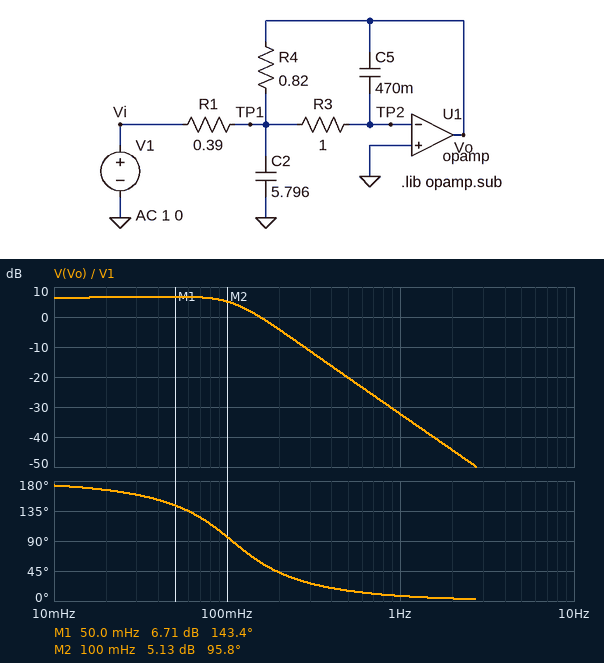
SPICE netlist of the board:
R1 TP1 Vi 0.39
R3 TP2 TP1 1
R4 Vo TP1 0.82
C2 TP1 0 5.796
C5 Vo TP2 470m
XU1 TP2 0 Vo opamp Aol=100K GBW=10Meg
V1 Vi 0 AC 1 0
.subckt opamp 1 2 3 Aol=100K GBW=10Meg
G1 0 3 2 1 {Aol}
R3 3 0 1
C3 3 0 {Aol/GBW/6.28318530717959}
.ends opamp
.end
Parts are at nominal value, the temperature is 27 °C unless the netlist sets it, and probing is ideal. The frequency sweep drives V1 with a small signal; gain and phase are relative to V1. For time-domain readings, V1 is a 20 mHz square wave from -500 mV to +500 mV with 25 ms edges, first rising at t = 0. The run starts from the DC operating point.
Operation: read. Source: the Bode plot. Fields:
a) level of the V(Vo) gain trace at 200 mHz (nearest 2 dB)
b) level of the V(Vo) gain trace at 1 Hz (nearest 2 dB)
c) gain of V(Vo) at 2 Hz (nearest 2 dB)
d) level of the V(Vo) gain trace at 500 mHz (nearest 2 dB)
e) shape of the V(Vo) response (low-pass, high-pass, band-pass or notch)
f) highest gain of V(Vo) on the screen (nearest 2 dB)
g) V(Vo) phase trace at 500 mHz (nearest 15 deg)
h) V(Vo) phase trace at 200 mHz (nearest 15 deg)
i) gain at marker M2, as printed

-4 dB
-32 dB
-44 dB
-20 dB
low-pass
6 dB
15 deg
45 deg
5.13 dB
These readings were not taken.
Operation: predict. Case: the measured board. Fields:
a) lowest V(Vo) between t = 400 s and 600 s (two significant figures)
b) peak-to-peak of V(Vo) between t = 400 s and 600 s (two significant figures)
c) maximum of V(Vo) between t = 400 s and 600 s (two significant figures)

-1.2 V
2.5 V
1.2 V
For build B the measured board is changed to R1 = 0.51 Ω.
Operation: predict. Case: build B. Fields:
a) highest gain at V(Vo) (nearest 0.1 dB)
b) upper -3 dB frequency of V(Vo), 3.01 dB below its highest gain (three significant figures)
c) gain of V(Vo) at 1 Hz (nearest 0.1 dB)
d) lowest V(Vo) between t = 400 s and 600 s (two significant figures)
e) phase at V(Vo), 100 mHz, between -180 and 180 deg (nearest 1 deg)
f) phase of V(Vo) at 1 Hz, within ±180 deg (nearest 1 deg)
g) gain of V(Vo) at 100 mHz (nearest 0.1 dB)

5.0 dB
123 mHz
-34.7 dB
-1.0 V
97 deg
7 deg
4.0 dB
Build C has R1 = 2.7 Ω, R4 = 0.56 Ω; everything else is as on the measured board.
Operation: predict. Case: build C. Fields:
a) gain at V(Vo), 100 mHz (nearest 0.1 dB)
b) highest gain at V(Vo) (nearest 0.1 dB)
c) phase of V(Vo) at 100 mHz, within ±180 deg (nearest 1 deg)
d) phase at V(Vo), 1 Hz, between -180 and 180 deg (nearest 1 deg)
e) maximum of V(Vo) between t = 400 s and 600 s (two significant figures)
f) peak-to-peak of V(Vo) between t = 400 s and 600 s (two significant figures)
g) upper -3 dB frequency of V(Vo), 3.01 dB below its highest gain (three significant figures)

-10.0 dB
-9.7 dB
127 deg
5 deg
170 mV
340 mV
153 mHz
